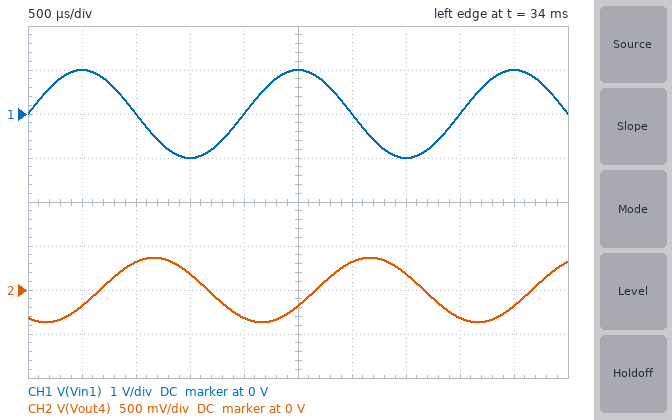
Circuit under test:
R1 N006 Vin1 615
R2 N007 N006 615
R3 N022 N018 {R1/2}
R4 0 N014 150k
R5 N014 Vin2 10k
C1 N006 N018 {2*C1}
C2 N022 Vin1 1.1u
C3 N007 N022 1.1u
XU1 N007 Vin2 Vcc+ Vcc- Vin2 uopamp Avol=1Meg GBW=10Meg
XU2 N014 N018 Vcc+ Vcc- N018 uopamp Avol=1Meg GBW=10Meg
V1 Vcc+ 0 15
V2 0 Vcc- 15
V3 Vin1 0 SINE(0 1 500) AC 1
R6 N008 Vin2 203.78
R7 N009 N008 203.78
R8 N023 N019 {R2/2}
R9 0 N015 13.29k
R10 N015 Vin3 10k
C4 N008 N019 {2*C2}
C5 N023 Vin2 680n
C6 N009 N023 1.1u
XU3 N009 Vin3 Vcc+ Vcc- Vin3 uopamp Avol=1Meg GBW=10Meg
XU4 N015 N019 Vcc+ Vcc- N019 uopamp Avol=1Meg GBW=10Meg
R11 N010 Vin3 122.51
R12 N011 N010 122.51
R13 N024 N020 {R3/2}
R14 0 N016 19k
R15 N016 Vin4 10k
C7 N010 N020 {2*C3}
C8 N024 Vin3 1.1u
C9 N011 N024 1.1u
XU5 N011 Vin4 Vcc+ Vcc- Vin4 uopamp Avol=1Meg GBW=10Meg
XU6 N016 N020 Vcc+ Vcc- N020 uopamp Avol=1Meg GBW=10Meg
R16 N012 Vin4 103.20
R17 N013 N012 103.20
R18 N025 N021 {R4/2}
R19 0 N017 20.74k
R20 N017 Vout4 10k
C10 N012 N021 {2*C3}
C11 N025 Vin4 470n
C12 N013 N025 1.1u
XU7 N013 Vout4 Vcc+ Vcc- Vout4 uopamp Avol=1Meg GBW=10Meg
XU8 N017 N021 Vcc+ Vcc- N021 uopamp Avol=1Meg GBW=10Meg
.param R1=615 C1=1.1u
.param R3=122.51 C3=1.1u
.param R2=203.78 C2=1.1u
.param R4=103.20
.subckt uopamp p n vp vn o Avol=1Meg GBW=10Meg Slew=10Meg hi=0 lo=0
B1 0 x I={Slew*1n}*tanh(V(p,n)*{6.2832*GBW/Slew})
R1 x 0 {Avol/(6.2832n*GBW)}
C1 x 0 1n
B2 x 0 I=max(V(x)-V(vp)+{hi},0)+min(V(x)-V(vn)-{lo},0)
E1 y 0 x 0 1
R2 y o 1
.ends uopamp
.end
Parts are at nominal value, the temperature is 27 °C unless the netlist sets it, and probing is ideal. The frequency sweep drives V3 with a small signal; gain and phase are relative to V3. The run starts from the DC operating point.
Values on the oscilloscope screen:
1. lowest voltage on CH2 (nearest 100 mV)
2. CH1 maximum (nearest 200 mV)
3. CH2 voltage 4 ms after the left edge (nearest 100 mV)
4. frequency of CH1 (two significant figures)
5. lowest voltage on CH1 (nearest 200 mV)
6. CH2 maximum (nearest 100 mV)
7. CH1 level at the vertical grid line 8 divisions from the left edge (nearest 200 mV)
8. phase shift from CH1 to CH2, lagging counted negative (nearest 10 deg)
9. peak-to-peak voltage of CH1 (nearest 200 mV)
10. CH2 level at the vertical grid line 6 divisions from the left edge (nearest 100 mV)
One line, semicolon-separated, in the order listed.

-400 mV; 1.0 V; -300 mV; 500 Hz; -1.0 V; 400 mV; 0 V; -120 deg; 2.0 V; 300 mV
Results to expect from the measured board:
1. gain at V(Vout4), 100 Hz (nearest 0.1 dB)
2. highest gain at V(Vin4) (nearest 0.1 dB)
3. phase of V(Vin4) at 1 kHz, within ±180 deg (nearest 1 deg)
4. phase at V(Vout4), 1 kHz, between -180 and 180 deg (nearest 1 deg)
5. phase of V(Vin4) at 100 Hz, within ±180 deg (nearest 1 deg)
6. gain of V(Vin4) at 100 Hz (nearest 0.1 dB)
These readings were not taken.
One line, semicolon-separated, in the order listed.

-0.4 dB; 0 dB; 25 deg; -31 deg; -28 deg; -0.4 dB
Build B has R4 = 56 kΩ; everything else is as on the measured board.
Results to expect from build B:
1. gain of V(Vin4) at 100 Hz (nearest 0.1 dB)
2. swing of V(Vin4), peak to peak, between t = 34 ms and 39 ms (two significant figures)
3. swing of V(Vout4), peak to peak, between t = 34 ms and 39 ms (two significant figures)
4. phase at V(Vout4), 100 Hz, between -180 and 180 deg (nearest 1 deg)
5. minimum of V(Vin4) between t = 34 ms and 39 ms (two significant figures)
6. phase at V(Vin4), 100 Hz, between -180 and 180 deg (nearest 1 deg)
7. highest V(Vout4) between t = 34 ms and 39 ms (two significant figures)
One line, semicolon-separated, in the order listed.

-0.7 dB; 760 mV; 700 mV; -43 deg; -380 mV; -38 deg; 350 mV
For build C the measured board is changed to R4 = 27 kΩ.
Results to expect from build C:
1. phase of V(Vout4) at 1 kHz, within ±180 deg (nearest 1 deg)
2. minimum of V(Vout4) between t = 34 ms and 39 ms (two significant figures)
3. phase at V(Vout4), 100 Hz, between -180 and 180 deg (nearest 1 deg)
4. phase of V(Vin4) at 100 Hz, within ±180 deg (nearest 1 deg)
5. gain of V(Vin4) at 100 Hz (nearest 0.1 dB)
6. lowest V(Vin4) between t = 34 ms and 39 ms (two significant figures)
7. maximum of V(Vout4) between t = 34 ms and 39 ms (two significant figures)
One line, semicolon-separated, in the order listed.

-20 deg; -310 mV; -55 deg; -50 deg; -1.5 dB; -340 mV; 310 mV
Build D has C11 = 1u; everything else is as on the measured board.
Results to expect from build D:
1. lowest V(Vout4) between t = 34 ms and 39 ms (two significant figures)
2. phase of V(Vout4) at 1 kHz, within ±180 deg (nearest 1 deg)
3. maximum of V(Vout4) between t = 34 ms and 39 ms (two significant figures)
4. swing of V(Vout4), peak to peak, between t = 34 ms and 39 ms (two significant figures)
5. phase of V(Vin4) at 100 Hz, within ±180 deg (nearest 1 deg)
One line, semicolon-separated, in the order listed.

-360 mV; -37 deg; 360 mV; 710 mV; -28 deg
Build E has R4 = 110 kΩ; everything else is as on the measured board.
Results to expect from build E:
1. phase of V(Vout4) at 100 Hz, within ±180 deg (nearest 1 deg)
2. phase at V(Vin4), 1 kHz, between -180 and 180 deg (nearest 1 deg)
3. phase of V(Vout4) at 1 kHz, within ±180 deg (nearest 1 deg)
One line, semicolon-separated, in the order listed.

-36 deg; 26 deg; -30 deg
